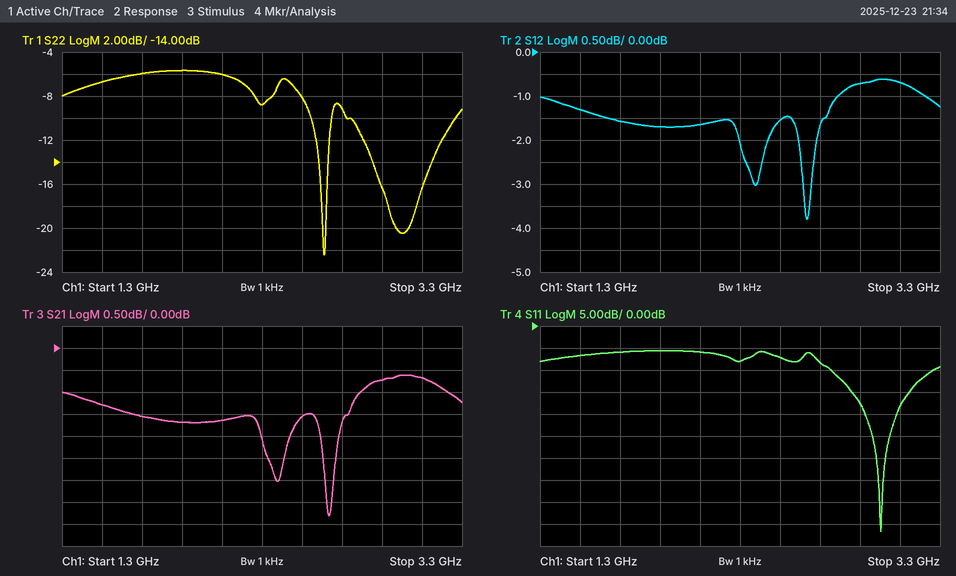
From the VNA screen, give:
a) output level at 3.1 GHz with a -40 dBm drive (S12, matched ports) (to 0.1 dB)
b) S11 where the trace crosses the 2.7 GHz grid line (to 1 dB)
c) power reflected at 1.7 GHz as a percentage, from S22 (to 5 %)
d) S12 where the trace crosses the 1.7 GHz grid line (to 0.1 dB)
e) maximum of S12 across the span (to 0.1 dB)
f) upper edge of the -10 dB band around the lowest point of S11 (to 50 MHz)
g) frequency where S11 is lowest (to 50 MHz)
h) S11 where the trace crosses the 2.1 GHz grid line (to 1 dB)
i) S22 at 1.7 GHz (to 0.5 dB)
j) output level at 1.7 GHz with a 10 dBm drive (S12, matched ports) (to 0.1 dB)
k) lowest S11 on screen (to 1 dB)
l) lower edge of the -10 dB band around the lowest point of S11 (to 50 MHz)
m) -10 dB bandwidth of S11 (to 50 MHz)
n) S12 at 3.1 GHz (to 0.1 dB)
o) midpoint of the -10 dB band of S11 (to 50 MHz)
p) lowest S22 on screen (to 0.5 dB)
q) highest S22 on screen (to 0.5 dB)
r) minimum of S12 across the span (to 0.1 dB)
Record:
-40.7 dBm
-8 dB
25 %
-1.6 dB
-0.6 dB
3.25 GHz
3.00 GHz
-6 dB
-6.0 dB
8.4 dBm
-47 dB
2.75 GHz
500 MHz
-0.7 dB
3.00 GHz
-22.5 dB
-5.5 dB
-3.8 dB
